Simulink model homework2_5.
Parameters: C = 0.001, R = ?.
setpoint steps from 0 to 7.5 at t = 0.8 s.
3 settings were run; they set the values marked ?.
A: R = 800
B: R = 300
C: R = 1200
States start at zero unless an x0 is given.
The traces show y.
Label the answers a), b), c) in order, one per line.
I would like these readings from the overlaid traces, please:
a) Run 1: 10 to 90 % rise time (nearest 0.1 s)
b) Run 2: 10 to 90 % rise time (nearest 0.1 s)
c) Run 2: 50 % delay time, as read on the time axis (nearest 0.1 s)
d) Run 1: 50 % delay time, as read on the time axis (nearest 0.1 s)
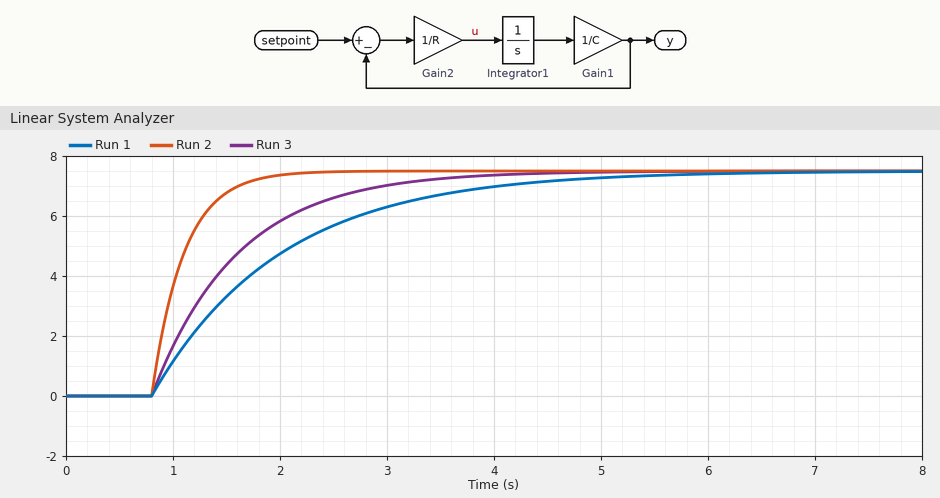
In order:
a) 2.6 s
b) 0.7 s
c) 1.0 s
d) 1.6 s
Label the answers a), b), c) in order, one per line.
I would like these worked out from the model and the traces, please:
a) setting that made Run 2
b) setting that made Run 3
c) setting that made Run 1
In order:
a) B
b) A
c) C
